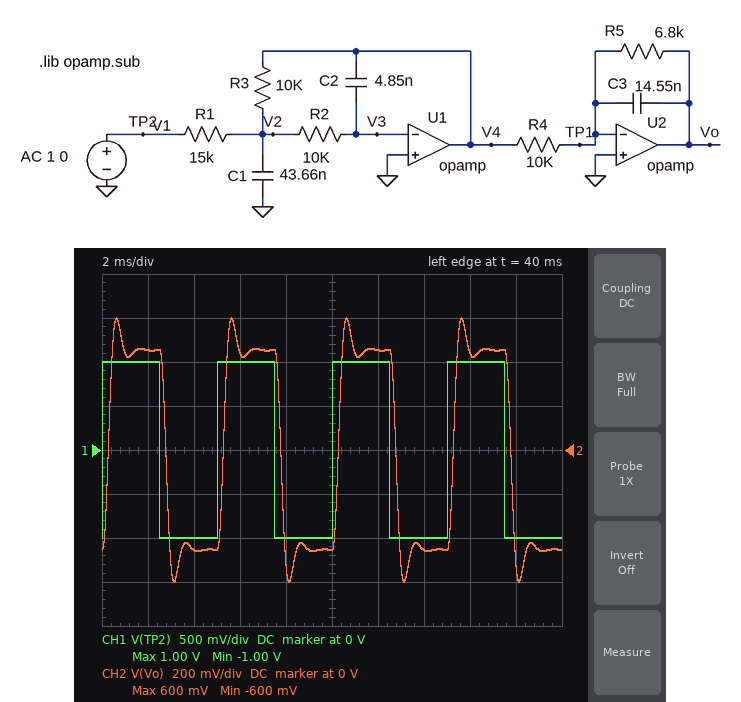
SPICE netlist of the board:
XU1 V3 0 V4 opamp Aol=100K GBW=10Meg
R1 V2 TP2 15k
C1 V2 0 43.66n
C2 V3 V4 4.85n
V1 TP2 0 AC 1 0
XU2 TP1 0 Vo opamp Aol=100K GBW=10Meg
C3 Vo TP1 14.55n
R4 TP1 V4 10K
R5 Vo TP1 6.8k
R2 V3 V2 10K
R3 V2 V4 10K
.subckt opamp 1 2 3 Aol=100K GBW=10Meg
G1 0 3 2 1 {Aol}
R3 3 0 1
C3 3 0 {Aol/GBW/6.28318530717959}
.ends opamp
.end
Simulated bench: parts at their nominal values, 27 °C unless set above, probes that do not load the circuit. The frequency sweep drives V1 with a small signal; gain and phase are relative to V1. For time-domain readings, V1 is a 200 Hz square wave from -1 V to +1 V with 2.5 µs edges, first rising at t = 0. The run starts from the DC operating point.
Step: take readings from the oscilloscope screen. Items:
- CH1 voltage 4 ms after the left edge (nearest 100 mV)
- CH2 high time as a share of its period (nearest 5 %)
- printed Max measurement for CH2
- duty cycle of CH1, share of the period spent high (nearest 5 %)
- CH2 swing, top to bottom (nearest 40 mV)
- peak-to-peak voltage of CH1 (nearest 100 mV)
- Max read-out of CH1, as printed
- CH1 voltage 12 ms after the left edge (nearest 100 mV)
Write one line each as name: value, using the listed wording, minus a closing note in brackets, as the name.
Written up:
CH1 voltage 4 ms after the left edge: -1.0 V
CH2 high time as a share of its period: 50 %
printed Max measurement for CH2: 600 mV
duty cycle of CH1, share of the period spent high: 50 %
CH2 swing, top to bottom: 1.20 V
peak-to-peak voltage of CH1: 2.0 V
Max read-out of CH1, as printed: 1.00 V
CH1 voltage 12 ms after the left edge: 1.0 V
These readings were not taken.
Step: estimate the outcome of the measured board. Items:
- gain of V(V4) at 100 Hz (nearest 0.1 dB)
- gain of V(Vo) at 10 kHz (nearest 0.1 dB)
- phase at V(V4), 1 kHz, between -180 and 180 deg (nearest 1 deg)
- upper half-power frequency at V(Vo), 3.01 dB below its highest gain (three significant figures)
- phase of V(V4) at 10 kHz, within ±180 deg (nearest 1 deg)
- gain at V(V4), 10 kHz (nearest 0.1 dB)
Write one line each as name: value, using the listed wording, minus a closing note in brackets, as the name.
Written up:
gain of V(V4) at 100 Hz: -3.5 dB
gain of V(Vo) at 10 kHz: -61.2 dB
phase at V(V4), 1 kHz, between -180 and 180 deg: 101 deg
upper half-power frequency at V(Vo), 3.01 dB below its highest gain: 1.21 kHz
phase of V(V4) at 10 kHz, within ±180 deg: 6 deg
gain at V(V4), 10 kHz: -41.9 dB
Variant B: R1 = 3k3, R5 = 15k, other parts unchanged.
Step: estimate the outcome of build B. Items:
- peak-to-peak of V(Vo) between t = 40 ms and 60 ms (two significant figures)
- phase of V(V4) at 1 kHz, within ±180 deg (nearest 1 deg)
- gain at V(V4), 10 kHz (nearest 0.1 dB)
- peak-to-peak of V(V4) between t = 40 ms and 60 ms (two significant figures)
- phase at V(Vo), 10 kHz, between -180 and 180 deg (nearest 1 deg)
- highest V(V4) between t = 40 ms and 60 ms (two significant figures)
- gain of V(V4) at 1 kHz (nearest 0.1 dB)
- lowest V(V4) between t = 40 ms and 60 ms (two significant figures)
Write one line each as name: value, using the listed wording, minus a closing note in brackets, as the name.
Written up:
peak-to-peak of V(Vo) between t = 40 ms and 60 ms: 9.1 V
phase of V(V4) at 1 kHz, within ±180 deg: 96 deg
gain at V(V4), 10 kHz: -28.9 dB
peak-to-peak of V(V4) between t = 40 ms and 60 ms: 6.2 V
phase at V(Vo), 10 kHz, between -180 and 180 deg: 105 deg
highest V(V4) between t = 40 ms and 60 ms: 3.1 V
gain of V(V4) at 1 kHz: 5.9 dB
lowest V(V4) between t = 40 ms and 60 ms: -3.1 V
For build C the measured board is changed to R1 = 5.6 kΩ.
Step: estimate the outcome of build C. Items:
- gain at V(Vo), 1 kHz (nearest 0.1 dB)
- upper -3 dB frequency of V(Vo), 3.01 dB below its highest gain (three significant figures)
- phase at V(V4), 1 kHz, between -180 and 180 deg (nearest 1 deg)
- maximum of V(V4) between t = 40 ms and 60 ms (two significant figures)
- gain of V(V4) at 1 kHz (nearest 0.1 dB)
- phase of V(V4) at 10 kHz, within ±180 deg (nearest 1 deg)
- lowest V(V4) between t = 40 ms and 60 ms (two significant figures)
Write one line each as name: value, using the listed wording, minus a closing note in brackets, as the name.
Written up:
gain at V(Vo), 1 kHz: -1.1 dB
upper -3 dB frequency of V(Vo), 3.01 dB below its highest gain: 1.03 kHz
phase at V(V4), 1 kHz, between -180 and 180 deg: 98 deg
maximum of V(V4) between t = 40 ms and 60 ms: 2.1 V
gain of V(V4) at 1 kHz: 3.7 dB
phase of V(V4) at 10 kHz, within ±180 deg: 8 deg
lowest V(V4) between t = 40 ms and 60 ms: -2.1 V
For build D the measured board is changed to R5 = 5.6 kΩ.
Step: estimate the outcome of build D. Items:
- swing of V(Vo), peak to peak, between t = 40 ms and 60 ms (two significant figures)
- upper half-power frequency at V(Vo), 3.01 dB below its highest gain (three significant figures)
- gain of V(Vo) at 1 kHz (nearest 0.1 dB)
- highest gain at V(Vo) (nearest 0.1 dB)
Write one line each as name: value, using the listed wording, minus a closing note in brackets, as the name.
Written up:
swing of V(Vo), peak to peak, between t = 40 ms and 60 ms: 1.0 V
upper half-power frequency at V(Vo), 3.01 dB below its highest gain: 1.23 kHz
gain of V(Vo) at 1 kHz: -7.9 dB
highest gain at V(Vo): -7.3 dB
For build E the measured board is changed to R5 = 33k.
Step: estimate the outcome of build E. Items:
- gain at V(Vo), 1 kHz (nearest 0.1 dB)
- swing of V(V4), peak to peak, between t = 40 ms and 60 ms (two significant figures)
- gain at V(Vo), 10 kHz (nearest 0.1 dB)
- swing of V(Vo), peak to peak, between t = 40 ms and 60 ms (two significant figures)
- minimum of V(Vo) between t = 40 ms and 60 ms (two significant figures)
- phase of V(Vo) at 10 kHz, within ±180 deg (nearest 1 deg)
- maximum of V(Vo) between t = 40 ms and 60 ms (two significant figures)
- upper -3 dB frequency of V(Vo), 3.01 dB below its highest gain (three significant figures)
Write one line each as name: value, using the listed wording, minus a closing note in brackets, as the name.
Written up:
gain at V(Vo), 1 kHz: -1.6 dB
swing of V(V4), peak to peak, between t = 40 ms and 60 ms: 1.9 V
gain at V(Vo), 10 kHz: -61.1 dB
swing of V(Vo), peak to peak, between t = 40 ms and 60 ms: 4.3 V
minimum of V(Vo) between t = 40 ms and 60 ms: -2.2 V
phase of V(Vo) at 10 kHz, within ±180 deg: 97 deg
maximum of V(Vo) between t = 40 ms and 60 ms: 2.2 V
upper -3 dB frequency of V(Vo), 3.01 dB below its highest gain: 378 Hz
